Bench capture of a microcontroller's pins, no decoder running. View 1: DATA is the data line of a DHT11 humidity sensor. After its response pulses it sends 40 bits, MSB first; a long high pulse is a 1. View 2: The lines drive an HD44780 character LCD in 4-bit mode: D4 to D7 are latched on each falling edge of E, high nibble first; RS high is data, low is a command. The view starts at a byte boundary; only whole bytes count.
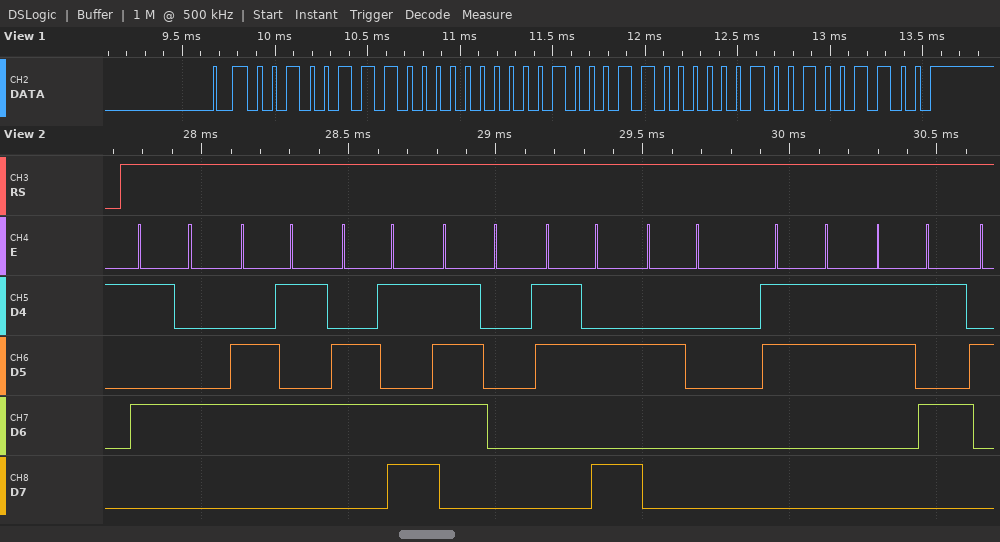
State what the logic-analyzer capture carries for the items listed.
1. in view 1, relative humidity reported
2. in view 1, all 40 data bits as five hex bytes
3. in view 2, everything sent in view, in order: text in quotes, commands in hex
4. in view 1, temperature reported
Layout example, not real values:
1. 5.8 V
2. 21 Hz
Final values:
1. 39 %
2. 27 00 23 02 4C
3. "Temp: 35"
4. 35.2 °C
